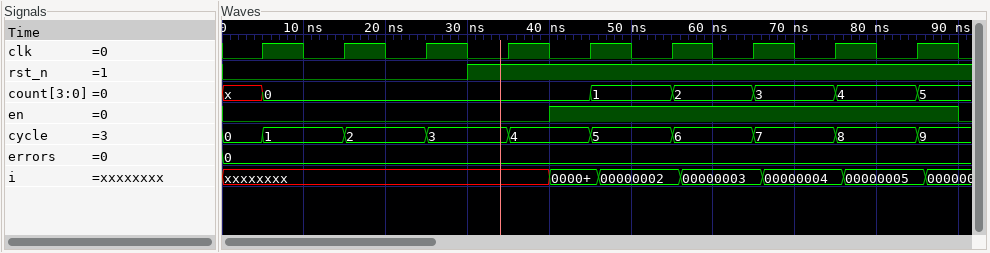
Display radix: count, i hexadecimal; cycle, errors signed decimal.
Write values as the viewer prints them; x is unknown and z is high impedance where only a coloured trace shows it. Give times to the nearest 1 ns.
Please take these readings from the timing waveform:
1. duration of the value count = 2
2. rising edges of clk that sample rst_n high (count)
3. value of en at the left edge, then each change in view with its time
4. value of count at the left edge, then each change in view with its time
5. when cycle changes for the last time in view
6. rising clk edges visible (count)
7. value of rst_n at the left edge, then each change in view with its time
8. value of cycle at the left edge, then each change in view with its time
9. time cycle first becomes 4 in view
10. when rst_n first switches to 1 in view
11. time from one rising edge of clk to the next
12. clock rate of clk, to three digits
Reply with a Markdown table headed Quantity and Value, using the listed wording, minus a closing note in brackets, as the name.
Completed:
| Quantity | Value |
|---|---|
| duration of the value count = 2 | 10 ns |
| rising edges of clk that sample rst_n high | 6 |
| value of en at the left edge, then each change in view with its time | 0, 1 at 40 ns, 0 at 90 ns |
| value of count at the left edge, then each change in view with its time | x, 0 at 5 ns, 1 at 45 ns, 2 at 55 ns, 3 at 65 ns, 4 at 75 ns, 5 at 85 ns |
| when cycle changes for the last time in view | 85 ns |
| rising clk edges visible | 9 |
| value of rst_n at the left edge, then each change in view with its time | 0, 1 at 30 ns |
| value of cycle at the left edge, then each change in view with its time | 0, 1 at 5 ns, 2 at 15 ns, 3 at 25 ns, 4 at 35 ns, 5 at 45 ns, 6 at 55 ns, 7 at 65 ns, 8 at 75 ns, 9 at 85 ns |
| time cycle first becomes 4 in view | 35 ns |
| when rst_n first switches to 1 in view | 30 ns |
| time from one rising edge of clk to the next | 10 ns |
| clock rate of clk, to three digits | 100 MHz |
